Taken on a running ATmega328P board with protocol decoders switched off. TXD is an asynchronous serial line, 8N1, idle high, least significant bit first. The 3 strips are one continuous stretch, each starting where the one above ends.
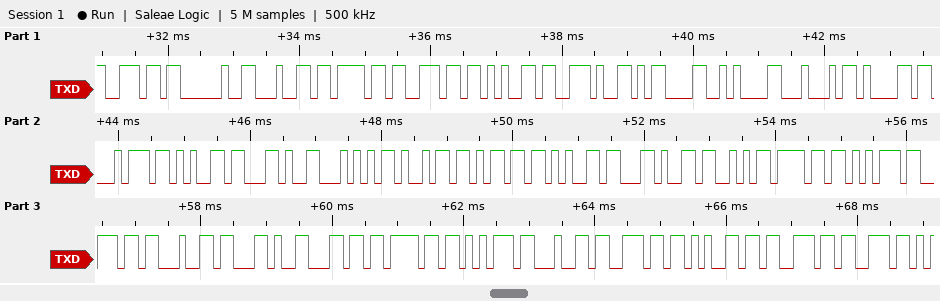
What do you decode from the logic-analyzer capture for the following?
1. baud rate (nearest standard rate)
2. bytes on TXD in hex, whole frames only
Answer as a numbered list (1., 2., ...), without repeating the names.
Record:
1. 9600 baud
2. 0x6E 0x20 0x64 0x6F 0x6E 0x65 0x2E 0x0D 0x0A 0x44 0x61 0x74 0x65 0x2C 0x54 0x69 0x6D 0x65 0x2C 0x53 0x6F 0x75 0x6E 0x64 0x2C 0x6C 0x6F 0x75 0x64 0x6E 0x65 0x73 0x73
